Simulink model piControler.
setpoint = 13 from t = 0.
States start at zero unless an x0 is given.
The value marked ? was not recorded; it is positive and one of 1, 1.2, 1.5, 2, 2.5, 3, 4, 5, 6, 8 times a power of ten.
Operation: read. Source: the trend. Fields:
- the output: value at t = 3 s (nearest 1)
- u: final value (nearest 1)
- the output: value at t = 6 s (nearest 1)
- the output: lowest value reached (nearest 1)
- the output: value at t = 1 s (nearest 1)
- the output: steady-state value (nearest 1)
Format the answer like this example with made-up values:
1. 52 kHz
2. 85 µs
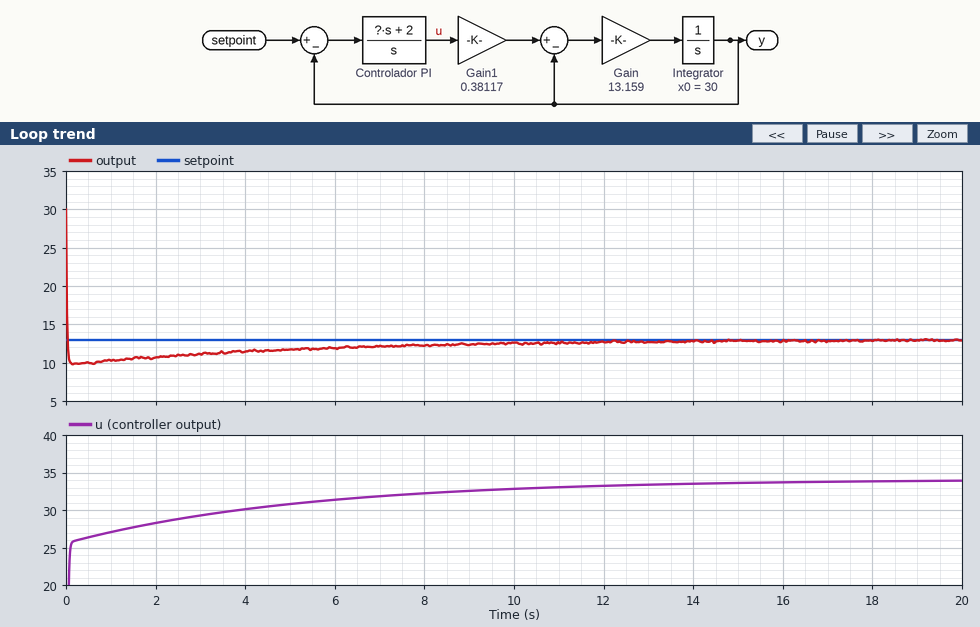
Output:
1. 11
2. 34
3. 12
4. 10
5. 10
6. 13
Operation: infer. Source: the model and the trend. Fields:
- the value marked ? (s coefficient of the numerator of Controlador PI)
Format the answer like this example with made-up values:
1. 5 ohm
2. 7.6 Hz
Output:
1. 8
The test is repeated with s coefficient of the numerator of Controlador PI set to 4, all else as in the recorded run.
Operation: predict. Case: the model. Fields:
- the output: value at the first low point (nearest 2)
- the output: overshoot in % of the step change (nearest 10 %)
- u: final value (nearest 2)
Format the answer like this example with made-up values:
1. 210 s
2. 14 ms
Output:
1. 8
2. 30 %
3. 34
